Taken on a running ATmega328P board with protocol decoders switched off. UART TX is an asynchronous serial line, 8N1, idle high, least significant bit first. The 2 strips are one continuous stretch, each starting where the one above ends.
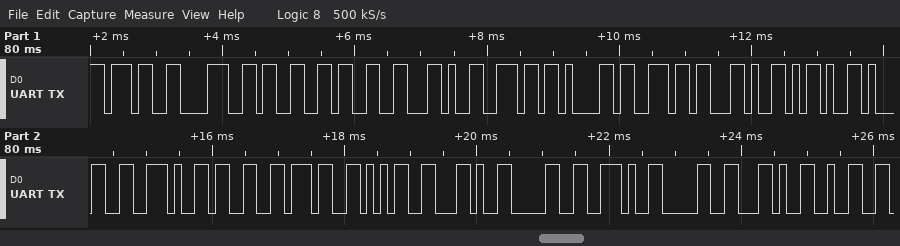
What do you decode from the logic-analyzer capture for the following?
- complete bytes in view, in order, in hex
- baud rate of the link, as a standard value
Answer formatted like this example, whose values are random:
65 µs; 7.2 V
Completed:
37 38 33 33 2C 6E 61 6E 2C 2D 31 2E 33 37 35 2C 30 2E 30 2C 32; 9600 baud
